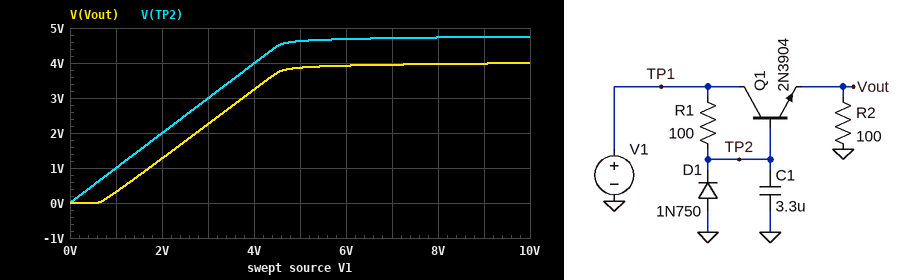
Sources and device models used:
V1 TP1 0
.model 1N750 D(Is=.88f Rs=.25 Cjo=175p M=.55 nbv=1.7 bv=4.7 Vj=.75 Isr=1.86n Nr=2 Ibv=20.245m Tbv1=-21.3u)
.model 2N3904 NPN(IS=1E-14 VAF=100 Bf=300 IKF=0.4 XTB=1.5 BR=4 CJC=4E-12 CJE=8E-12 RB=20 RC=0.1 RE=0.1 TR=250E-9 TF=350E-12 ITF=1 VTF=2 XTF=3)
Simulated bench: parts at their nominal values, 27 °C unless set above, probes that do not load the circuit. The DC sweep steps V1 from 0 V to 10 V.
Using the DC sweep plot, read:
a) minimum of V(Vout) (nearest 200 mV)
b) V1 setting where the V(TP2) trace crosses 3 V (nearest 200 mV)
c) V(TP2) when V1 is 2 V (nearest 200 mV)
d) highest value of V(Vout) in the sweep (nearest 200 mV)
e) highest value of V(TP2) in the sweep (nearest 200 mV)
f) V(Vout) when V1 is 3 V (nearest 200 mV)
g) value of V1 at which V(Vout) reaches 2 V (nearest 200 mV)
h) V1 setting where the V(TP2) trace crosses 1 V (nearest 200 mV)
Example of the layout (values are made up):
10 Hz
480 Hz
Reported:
0 V
3.0 V
2.0 V
4.0 V
4.8 V
2.2 V
2.8 V
1.0 V
